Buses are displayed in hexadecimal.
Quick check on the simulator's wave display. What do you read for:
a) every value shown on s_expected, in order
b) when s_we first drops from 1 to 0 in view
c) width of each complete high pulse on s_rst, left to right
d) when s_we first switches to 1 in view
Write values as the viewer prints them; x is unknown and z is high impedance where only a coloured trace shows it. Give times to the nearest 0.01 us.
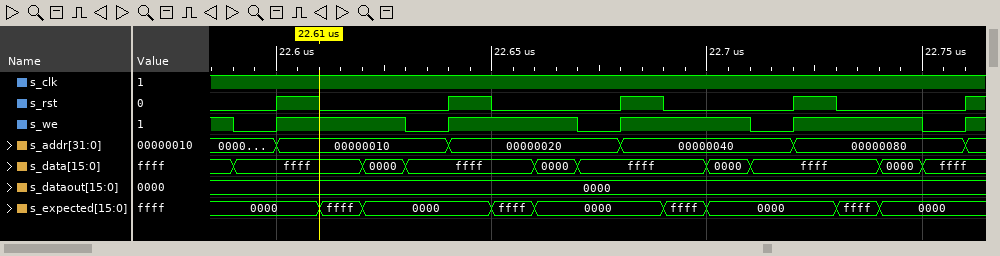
0000, ffff, 0000, ffff, 0000, ffff, 0000, ffff, 0000
22.59 us
0.01 us, 0.01 us, 0.01 us, 0.01 us
22.6 us
